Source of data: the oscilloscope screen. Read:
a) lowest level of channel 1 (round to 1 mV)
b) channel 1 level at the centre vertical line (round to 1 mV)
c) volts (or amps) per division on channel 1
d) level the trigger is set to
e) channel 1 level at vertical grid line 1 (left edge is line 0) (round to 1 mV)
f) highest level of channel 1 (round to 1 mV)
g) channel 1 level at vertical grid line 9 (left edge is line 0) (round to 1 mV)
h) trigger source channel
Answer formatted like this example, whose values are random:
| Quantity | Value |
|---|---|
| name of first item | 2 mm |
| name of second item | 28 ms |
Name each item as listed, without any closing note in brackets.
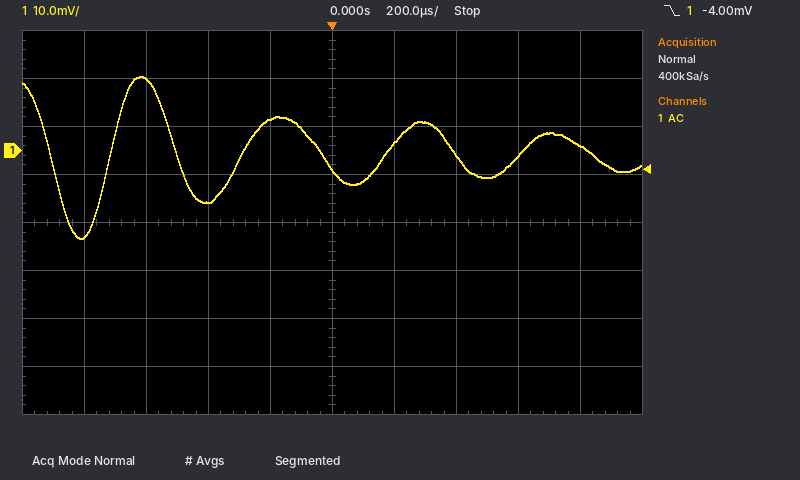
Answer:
| Quantity | Value |
|---|---|
| lowest level of channel 1 | -18 mV |
| channel 1 level at the centre vertical line | -4 mV |
| volts (or amps) per division on channel 1 | 10 mV |
| level the trigger is set to | -4.00 mV |
| channel 1 level at vertical grid line 1 (left edge is line 0) | -18 mV |
| highest level of channel 1 | 15 mV |
| channel 1 level at vertical grid line 9 (left edge is line 0) | 1 mV |
| trigger source channel | channel 1 |
